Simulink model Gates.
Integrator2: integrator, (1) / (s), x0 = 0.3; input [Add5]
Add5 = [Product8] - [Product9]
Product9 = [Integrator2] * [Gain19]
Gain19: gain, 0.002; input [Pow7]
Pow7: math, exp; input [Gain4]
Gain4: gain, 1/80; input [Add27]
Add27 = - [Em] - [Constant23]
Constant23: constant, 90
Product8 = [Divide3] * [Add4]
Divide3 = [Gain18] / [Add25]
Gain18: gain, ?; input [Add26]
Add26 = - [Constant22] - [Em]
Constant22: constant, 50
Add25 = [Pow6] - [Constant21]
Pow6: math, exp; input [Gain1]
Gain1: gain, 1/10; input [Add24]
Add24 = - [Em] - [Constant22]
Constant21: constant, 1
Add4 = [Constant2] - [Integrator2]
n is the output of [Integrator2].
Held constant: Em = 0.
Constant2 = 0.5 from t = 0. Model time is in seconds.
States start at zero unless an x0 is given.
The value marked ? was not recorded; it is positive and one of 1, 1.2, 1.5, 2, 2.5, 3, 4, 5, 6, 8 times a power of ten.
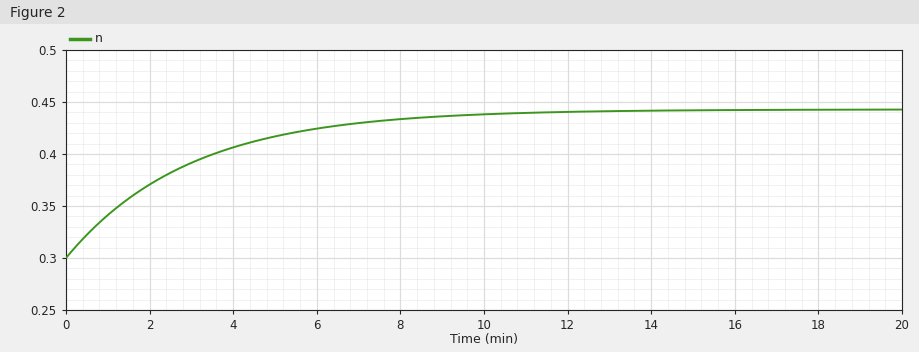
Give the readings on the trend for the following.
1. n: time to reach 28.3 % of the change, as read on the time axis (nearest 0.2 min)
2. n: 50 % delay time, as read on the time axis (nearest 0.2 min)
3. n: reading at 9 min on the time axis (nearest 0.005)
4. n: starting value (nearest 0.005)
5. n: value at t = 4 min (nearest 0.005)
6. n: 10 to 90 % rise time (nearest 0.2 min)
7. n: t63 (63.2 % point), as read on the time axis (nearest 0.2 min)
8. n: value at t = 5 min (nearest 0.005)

1.0 min
2.0 min
0.435
0.300
0.405
6.4 min
3.0 min
0.415
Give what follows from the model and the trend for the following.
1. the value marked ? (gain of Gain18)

0.0001
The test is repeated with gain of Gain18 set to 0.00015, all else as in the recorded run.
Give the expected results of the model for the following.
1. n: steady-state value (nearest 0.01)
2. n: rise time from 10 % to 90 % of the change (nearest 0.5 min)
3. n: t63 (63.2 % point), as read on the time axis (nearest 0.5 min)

0.46
4.5 min
2.0 min
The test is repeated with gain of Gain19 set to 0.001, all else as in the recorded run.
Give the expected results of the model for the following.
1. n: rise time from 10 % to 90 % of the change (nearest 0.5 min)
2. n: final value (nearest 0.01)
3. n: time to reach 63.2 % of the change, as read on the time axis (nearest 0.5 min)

7.0 min
0.47
3.0 min
